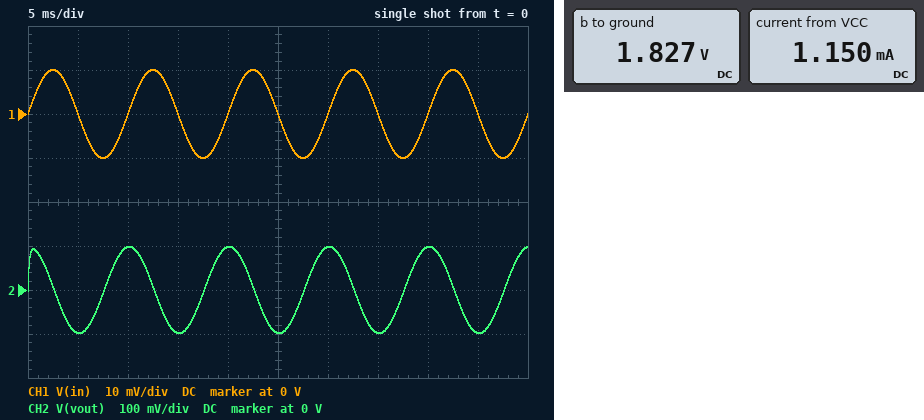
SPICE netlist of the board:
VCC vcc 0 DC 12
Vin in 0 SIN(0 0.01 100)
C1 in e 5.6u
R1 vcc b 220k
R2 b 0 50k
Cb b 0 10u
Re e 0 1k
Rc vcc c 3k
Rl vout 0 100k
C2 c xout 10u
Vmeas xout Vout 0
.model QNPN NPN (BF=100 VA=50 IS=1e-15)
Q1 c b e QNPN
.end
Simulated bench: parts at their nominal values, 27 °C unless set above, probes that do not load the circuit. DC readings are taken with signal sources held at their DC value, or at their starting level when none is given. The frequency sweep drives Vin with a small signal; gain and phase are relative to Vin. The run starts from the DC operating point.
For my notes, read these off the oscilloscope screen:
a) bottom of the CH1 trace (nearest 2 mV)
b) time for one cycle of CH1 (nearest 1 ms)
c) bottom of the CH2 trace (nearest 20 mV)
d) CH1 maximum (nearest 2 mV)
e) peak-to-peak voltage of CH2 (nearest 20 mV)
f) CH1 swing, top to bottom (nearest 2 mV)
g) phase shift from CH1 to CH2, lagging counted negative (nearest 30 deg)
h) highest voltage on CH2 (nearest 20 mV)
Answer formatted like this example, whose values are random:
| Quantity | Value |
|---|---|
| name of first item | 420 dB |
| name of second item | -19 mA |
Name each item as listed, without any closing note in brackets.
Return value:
| Quantity | Value |
|---|---|
| bottom of the CH1 trace | -10 mV |
| time for one cycle of CH1 | 10 ms |
| bottom of the CH2 trace | -100 mV |
| CH1 maximum | 10 mV |
| peak-to-peak voltage of CH2 | 200 mV |
| CH1 swing, top to bottom | 20 mV |
| phase shift from CH1 to CH2, lagging counted negative | 90 deg |
| highest voltage on CH2 | 100 mV |
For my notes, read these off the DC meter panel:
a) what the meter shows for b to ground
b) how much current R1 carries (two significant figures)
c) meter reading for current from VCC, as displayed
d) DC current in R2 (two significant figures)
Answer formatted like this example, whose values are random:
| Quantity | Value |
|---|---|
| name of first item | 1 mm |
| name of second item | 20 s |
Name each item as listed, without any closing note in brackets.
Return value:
| Quantity | Value |
|---|---|
| what the meter shows for b to ground | 1.827 V |
| how much current R1 carries | 46 µA |
| meter reading for current from VCC, as displayed | 1.150 mA |
| DC current in R2 | 37 µA |
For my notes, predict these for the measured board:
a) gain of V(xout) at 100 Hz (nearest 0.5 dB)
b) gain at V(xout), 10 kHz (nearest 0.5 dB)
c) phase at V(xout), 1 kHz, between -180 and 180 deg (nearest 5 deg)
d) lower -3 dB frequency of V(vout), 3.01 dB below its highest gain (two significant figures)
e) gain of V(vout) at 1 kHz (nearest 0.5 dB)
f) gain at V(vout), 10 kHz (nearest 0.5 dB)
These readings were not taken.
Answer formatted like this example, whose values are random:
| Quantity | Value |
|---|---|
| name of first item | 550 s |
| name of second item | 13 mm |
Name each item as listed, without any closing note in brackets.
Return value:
| Quantity | Value |
|---|---|
| gain of V(xout) at 100 Hz | 20.0 dB |
| gain at V(xout), 10 kHz | 41.5 dB |
| phase at V(xout), 1 kHz, between -180 and 180 deg | 50 deg |
| lower -3 dB frequency of V(vout), 3.01 dB below its highest gain | 1.2 kHz |
| gain of V(vout) at 1 kHz | 37.5 dB |
| gain at V(vout), 10 kHz | 41.5 dB |
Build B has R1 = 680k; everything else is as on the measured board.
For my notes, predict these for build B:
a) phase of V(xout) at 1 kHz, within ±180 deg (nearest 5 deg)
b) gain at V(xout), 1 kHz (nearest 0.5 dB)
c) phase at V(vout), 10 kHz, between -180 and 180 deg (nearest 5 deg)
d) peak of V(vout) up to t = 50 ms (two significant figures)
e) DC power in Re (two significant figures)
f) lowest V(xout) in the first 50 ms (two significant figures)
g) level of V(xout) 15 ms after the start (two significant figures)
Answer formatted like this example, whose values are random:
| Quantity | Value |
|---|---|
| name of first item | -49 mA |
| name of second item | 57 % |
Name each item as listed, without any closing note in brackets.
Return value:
| Quantity | Value |
|---|---|
| phase of V(xout) at 1 kHz, within ±180 deg | 10 deg |
| gain at V(xout), 1 kHz | 22.5 dB |
| phase at V(vout), 10 kHz, between -180 and 180 deg | 0 deg |
| peak of V(vout) up to t = 50 ms | 68 mV |
| DC power in Re | 15 µW |
| lowest V(xout) in the first 50 ms | -74 mV |
| level of V(xout) 15 ms after the start | -63 mV |
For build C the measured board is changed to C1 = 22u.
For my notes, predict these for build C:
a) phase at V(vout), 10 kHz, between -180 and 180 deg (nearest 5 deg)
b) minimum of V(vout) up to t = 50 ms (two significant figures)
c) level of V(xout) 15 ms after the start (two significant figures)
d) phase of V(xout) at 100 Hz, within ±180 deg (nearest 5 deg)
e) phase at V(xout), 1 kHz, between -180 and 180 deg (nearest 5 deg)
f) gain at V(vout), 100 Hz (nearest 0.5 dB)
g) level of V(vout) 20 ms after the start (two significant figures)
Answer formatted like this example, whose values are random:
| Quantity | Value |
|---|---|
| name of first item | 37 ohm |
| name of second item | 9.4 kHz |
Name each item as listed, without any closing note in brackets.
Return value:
| Quantity | Value |
|---|---|
| phase at V(vout), 10 kHz, between -180 and 180 deg | 0 deg |
| minimum of V(vout) up to t = 50 ms | -370 mV |
| level of V(xout) 15 ms after the start | -350 mV |
| phase of V(xout) at 100 Hz, within ±180 deg | 70 deg |
| phase at V(xout), 1 kHz, between -180 and 180 deg | 15 deg |
| gain at V(vout), 100 Hz | 31.0 dB |
| level of V(vout) 20 ms after the start | 340 mV |
